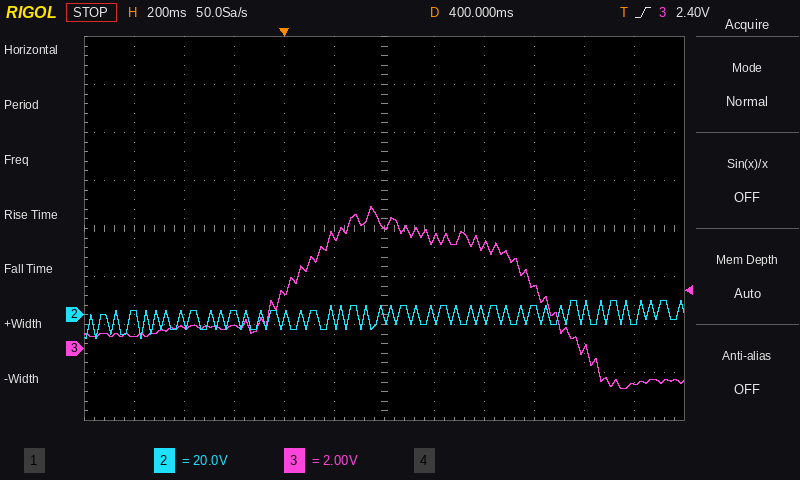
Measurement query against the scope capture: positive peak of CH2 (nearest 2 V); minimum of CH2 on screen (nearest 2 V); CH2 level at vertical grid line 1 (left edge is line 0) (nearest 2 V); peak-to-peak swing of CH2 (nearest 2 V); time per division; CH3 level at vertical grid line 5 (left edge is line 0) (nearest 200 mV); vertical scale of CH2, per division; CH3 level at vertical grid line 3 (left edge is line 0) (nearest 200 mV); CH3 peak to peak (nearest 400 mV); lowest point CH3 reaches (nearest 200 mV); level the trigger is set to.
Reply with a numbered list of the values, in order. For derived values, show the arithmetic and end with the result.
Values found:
1. 6 V
2. -10 V
3. 0 V
4. 6 V − (-10 V) = 16 V
5. 200 ms
6. 4.6 V
7. 20 V
8. 1.0 V
9. 7.6 V
10. -1.6 V
11. 2.40 V
